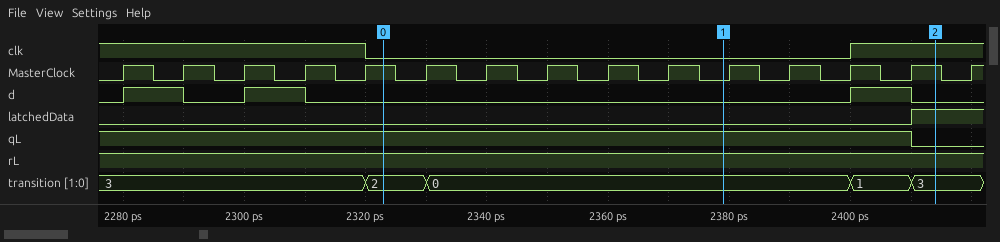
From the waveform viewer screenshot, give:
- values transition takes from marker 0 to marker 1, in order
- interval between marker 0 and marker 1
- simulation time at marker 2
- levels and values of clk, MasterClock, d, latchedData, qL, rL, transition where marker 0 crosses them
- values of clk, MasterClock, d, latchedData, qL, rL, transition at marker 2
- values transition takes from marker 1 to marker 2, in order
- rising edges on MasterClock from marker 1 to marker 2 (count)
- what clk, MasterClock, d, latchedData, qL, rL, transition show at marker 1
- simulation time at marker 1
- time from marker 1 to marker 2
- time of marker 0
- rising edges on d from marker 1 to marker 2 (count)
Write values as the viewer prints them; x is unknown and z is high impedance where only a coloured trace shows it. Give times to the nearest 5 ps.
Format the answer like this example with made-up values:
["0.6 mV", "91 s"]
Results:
["2, 0", "55 ps", "2415 ps", "clk=0, MasterClock=1, d=0, latchedData=0, qL=1, rL=1, transition=2", "clk=1, MasterClock=1, d=0, latchedData=1, qL=0, rL=1, transition=3", "0, 1, 3", "4", "clk=0, MasterClock=0, d=0, latchedData=0, qL=1, rL=1, transition=0", "2380 ps", "35 ps", "2325 ps", "1"]
